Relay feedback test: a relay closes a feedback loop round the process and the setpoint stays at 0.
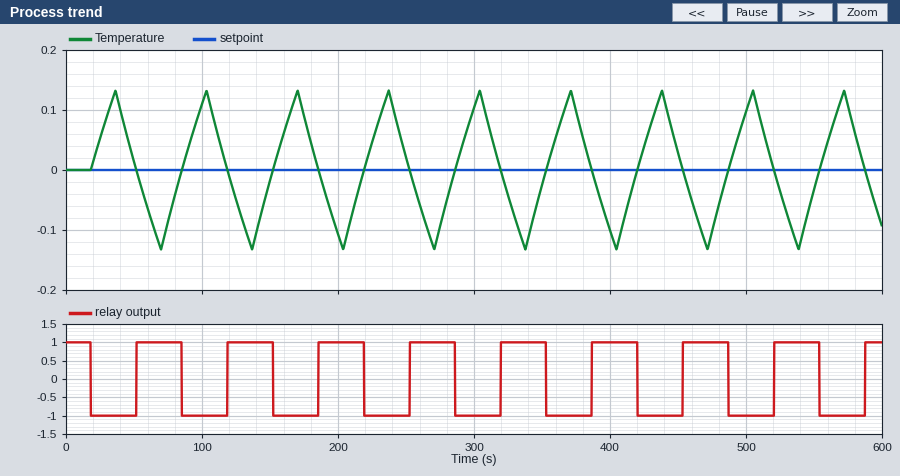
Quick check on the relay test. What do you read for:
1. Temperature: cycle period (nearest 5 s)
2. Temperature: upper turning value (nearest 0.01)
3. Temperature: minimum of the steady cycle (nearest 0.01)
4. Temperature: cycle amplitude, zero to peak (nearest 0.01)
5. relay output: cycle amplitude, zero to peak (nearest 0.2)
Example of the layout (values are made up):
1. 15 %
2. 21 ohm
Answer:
1. 65 s
2. 0.13
3. -0.13
4. 0.13
5. 1.0
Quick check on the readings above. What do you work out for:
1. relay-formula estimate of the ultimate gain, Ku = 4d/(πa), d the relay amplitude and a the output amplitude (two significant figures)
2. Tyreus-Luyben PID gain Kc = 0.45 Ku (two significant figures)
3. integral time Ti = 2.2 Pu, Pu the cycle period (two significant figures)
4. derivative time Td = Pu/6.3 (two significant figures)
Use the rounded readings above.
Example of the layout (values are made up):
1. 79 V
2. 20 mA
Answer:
1. 9.8
2. 4.4
3. 140 s
4. 10 s
